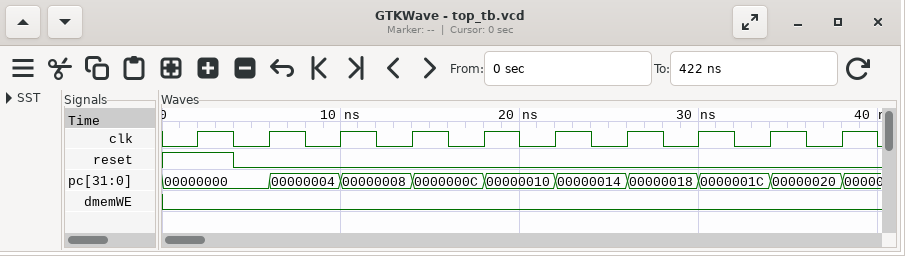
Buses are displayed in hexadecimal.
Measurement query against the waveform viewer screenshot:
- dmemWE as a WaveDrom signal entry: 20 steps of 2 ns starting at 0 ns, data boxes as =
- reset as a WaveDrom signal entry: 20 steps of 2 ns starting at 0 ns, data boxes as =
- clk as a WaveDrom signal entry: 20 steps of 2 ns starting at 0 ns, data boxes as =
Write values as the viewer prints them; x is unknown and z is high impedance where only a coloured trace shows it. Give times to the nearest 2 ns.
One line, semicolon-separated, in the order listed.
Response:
{name: 'dmemWE', wave: '0...................'}; {name: 'reset', wave: '1.0.................'}; {name: 'clk', wave: '01010101010101010101'}
